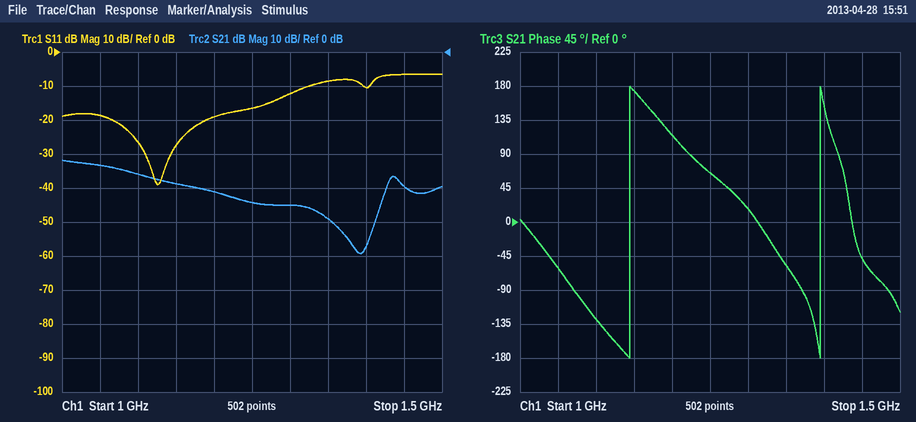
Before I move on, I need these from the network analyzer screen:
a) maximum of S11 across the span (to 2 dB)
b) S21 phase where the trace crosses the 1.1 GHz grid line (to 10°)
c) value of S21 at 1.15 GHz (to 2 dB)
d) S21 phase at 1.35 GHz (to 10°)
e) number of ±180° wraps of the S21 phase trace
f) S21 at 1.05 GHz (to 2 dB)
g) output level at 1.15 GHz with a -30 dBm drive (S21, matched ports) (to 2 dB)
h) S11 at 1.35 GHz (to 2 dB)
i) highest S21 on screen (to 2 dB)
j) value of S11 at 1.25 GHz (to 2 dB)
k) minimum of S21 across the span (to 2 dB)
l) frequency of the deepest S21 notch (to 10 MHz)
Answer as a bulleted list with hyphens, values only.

- -6 dB
- -130°
- -38 dB
- -60°
- 2
- -34 dB
- -68 dBm
- -8 dB
- -32 dB
- -16 dB
- -60 dB
- 1.39 GHz
